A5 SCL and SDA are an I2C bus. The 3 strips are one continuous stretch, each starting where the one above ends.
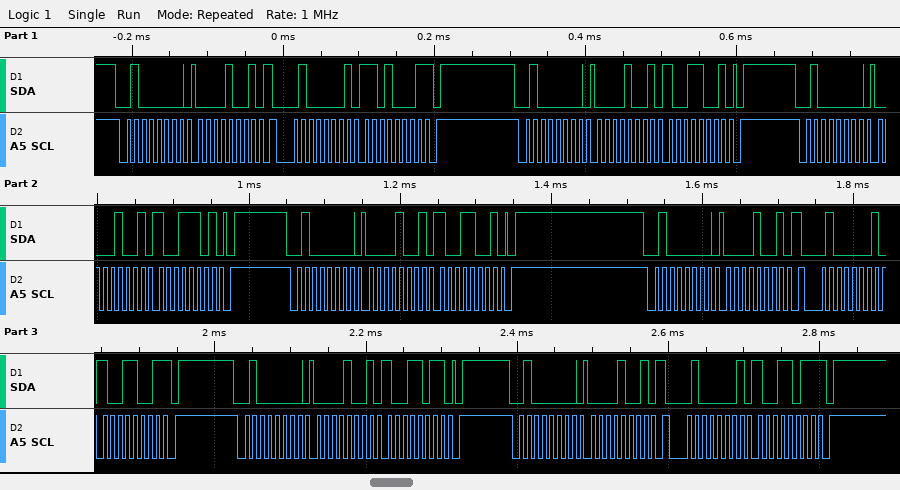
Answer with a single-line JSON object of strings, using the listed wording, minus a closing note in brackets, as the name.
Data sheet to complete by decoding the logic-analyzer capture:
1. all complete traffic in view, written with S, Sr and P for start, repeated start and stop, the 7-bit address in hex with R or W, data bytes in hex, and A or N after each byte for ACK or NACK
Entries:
{"all complete traffic in view, written with S, Sr and P for start, repeated start and stop, the 7-bit address in hex with R or W, data bytes in hex, and A or N after each byte for ACK or NACK": "S 20W A 09 A Sr 20R A D1 N P S 20W A 09 A 99 A P S 20W A 09 A 9D A P S 20W A 09 A 99 A P S 20W A 09 A Sr 20R A 99 N P S 20W A 09 A 9B A P S 20W A 09 A Sr 20R A 9B N P"}
